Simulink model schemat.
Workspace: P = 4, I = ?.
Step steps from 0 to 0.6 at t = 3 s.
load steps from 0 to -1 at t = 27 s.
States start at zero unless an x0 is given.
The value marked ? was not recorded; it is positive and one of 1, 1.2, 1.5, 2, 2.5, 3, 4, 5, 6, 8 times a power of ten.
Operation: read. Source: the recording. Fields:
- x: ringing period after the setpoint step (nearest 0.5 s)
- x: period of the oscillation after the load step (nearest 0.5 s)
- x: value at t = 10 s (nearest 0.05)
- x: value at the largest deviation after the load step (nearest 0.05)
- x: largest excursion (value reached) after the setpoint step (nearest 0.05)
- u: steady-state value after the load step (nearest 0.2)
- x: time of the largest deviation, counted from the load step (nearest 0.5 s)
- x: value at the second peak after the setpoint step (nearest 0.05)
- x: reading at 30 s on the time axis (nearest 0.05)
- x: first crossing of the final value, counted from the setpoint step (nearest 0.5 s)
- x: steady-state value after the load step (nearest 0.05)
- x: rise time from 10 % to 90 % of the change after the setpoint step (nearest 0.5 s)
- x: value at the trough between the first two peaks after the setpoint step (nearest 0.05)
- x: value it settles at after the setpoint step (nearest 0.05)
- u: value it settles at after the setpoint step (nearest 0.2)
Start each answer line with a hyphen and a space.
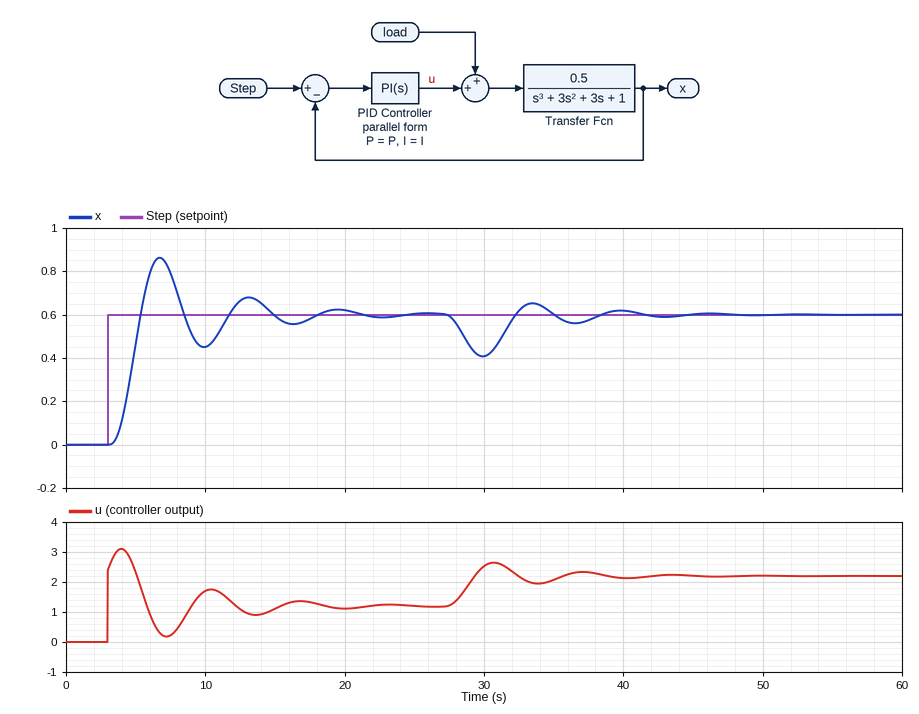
- 6.5 s
- 6.5 s
- 0.45
- 0.40
- 0.85
- 2.2
- 3.0 s
- 0.70
- 0.40
- 2.5 s
- 0.60
- 1.5 s
- 0.45
- 0.60
- 1.2
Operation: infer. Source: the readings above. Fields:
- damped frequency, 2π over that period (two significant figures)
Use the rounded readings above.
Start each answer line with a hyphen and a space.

- 0.97 rad/s
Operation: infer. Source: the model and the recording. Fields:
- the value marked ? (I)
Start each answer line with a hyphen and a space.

- 2
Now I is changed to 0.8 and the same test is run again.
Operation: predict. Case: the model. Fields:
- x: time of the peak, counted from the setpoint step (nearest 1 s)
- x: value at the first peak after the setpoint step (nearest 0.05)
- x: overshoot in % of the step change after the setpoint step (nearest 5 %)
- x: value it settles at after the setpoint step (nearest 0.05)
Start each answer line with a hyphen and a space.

- 4 s
- 0.65
- 10 %
- 0.60
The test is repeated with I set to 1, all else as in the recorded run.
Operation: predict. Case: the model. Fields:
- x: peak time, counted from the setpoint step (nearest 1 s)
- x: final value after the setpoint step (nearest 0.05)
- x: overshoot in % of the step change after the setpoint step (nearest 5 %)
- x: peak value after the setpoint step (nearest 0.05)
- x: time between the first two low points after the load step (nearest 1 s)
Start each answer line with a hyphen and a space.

- 4 s
- 0.60
- 15 %
- 0.70
- 6 s
